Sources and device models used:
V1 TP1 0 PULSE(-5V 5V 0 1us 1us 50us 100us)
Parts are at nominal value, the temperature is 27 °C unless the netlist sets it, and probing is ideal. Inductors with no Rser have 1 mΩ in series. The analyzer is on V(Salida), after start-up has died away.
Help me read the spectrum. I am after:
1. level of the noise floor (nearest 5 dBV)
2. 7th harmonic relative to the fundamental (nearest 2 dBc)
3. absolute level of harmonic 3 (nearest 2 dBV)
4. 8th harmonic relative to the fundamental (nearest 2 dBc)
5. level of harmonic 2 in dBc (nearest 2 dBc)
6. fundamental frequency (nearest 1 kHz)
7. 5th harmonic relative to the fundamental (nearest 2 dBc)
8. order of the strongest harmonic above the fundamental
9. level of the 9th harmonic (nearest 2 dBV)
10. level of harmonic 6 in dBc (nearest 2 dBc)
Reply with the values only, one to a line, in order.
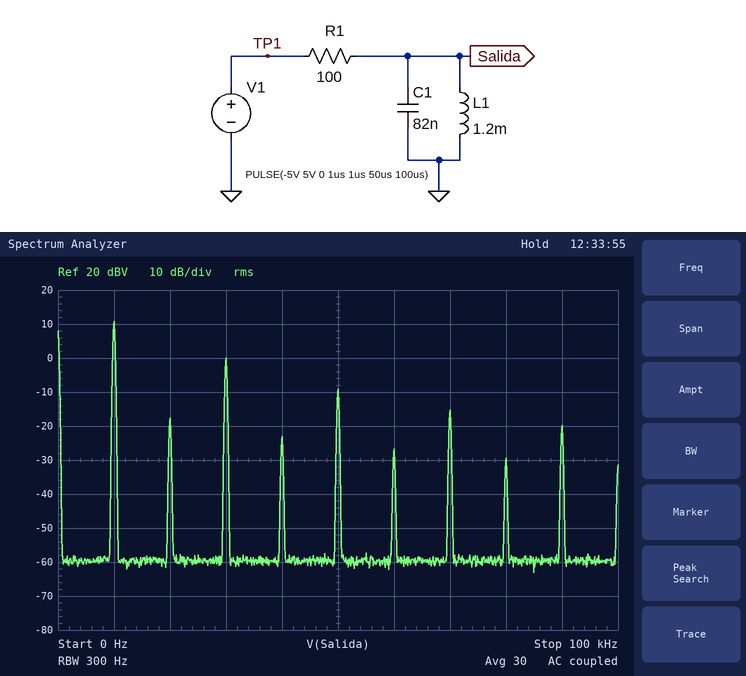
-60 dBV
-26 dBc
0 dBV
-40 dBc
-28 dBc
10 kHz
-20 dBc
3
-20 dBV
-38 dBc
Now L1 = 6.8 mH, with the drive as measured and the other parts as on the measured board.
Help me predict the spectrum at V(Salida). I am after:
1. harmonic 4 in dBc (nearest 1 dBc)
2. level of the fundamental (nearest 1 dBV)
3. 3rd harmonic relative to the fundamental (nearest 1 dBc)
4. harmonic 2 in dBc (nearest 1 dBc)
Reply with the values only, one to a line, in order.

-37 dBc
13 dBV
-14 dBc
-32 dBc
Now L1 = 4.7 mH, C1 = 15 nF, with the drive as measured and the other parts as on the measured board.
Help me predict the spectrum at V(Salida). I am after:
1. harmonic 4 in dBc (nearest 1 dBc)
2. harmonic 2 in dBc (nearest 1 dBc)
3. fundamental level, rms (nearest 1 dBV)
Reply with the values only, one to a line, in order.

-30 dBc
-30 dBc
13 dBV
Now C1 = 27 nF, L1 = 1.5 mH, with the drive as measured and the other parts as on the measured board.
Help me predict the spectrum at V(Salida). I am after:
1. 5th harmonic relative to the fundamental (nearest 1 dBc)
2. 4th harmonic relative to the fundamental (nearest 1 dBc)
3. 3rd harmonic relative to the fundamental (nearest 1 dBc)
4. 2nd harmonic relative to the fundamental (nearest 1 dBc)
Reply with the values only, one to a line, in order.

-13 dBc
-28 dBc
-7 dBc
-28 dBc
